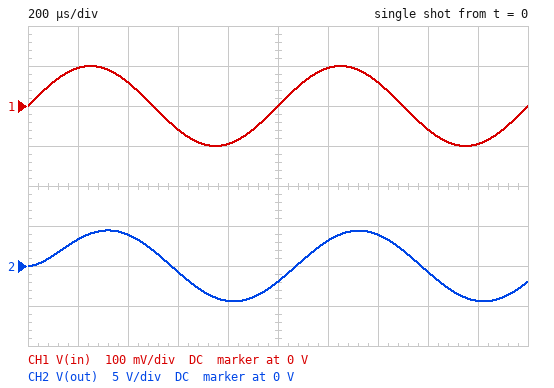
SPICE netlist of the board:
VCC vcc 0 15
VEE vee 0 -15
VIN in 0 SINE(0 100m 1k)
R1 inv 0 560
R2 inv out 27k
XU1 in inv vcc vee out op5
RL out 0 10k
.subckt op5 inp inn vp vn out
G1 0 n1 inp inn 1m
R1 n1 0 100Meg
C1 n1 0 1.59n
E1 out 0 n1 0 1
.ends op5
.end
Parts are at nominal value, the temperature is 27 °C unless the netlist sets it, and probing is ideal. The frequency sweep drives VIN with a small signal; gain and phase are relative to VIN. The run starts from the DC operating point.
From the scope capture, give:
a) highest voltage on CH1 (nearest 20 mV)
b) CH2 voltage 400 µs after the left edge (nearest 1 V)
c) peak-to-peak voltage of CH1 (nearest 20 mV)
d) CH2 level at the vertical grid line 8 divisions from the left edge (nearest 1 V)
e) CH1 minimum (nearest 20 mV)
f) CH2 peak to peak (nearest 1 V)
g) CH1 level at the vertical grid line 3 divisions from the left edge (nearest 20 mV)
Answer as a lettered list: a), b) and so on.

a) 100 mV
b) 4 V
c) 200 mV
d) -1 V
e) -100 mV
f) 9 V
g) -60 mV
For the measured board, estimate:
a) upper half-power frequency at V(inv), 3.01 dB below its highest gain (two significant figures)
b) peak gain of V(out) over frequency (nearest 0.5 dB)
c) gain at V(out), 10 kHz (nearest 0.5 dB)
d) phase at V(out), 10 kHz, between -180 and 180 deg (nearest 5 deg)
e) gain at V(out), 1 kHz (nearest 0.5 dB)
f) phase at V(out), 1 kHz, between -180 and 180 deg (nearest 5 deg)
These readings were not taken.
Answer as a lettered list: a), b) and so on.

a) 2.0 kHz
b) 34.0 dB
c) 20.0 dB
d) -80 deg
e) 33.0 dB
f) -25 deg
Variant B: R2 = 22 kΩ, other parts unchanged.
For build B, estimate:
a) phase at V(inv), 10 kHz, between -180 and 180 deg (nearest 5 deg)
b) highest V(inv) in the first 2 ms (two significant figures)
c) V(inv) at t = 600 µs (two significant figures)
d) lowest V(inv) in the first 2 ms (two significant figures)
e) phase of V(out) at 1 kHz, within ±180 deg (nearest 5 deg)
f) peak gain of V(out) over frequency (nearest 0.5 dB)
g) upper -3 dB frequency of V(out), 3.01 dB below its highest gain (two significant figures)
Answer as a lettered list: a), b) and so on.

a) -75 deg
b) 93 mV
c) -23 mV
d) -93 mV
e) -20 deg
f) 32.0 dB
g) 2.5 kHz
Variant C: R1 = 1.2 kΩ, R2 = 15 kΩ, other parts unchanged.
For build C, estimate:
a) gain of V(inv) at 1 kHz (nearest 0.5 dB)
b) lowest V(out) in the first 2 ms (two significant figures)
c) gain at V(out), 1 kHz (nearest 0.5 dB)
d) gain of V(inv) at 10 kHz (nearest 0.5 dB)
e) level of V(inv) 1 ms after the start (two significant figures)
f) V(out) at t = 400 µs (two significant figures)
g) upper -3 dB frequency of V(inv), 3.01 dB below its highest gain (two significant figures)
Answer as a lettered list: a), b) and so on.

a) 0 dB
b) -1.3 V
c) 22.5 dB
d) -4.5 dB
e) -13 mV
f) 920 mV
g) 7.4 kHz
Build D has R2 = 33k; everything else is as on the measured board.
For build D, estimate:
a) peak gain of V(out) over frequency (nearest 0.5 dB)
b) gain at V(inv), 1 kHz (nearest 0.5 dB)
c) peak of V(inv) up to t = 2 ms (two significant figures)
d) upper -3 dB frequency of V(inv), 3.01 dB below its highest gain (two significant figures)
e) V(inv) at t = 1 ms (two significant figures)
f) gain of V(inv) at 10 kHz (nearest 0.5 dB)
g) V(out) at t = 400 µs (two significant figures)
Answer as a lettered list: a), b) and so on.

a) 35.5 dB
b) -1.5 dB
c) 87 mV
d) 1.7 kHz
e) -44 mV
f) -15.5 dB
g) 4.8 V
